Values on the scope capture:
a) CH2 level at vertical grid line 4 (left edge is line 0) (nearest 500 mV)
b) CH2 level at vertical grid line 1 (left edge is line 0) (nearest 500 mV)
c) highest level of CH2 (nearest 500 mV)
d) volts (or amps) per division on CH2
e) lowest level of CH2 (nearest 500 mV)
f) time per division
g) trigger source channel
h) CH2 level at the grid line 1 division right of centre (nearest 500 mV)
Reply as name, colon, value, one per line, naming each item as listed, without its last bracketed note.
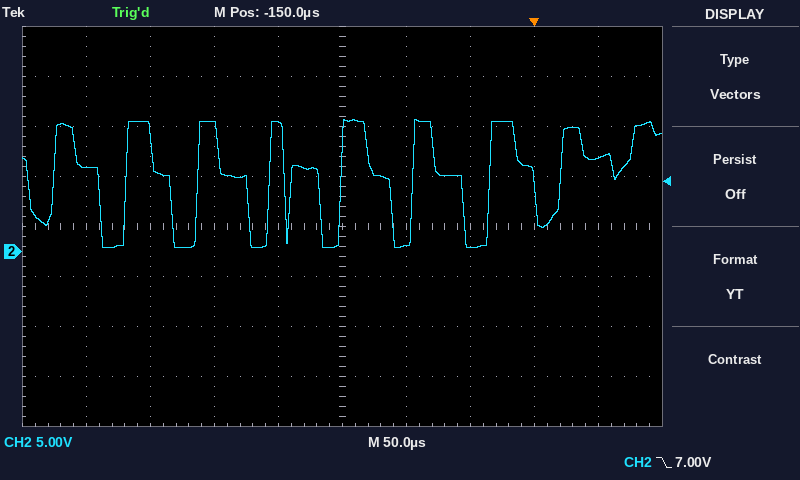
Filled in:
CH2 level at vertical grid line 4 (left edge is line 0): 13.0 V
CH2 level at vertical grid line 1 (left edge is line 0): 8.5 V
highest level of CH2: 13.0 V
volts (or amps) per division on CH2: 5 V
lowest level of CH2: 500 mV
time per division: 50 µs
trigger source channel: CH2
CH2 level at the grid line 1 division right of centre: 500 mV
